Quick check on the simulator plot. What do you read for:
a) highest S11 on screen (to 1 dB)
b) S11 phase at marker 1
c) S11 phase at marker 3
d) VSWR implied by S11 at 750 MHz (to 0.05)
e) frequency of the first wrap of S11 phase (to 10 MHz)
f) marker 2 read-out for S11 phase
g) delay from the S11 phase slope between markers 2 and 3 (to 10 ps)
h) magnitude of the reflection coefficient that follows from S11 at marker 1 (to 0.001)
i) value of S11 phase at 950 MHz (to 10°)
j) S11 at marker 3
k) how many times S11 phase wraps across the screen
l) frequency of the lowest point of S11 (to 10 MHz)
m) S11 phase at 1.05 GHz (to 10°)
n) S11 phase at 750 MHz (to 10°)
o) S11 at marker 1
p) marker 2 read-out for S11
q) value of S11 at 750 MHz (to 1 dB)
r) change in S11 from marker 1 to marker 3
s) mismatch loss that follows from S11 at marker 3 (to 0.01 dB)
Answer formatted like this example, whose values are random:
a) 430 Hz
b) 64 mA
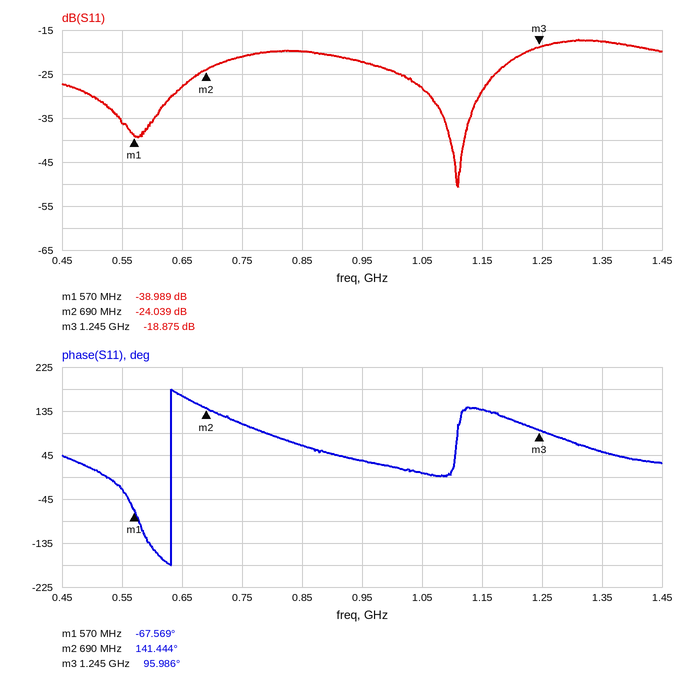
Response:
a) -17 dB
b) -67.569°
c) 95.986°
d) 1.20
e) 630 MHz
f) 141.444°
g) 230 ps
h) 0.011
i) 30°
j) -18.875 dB
k) 1
l) 1.11 GHz
m) 10°
n) 110°
o) -38.989 dB
p) -24.039 dB
q) -21 dB
r) 20.114 dB
s) 0.06 dB
